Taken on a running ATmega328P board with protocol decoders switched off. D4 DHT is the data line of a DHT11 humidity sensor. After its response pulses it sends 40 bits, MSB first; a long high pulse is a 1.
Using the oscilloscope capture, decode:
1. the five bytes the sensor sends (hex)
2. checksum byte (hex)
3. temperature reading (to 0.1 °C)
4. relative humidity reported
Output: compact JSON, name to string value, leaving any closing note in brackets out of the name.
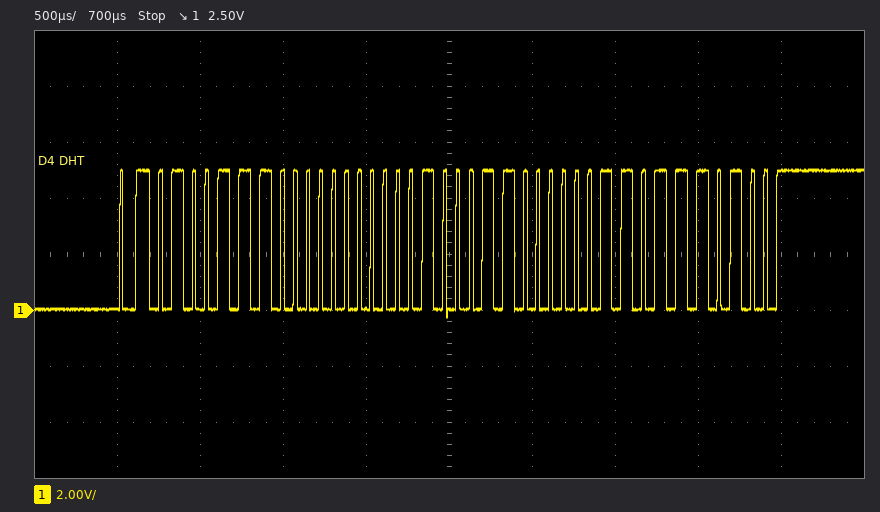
{"the five bytes the sensor sends": "4E 00 23 03 74", "checksum byte": "0x74", "temperature reading": "35.3 °C", "relative humidity reported": "78 %"}
